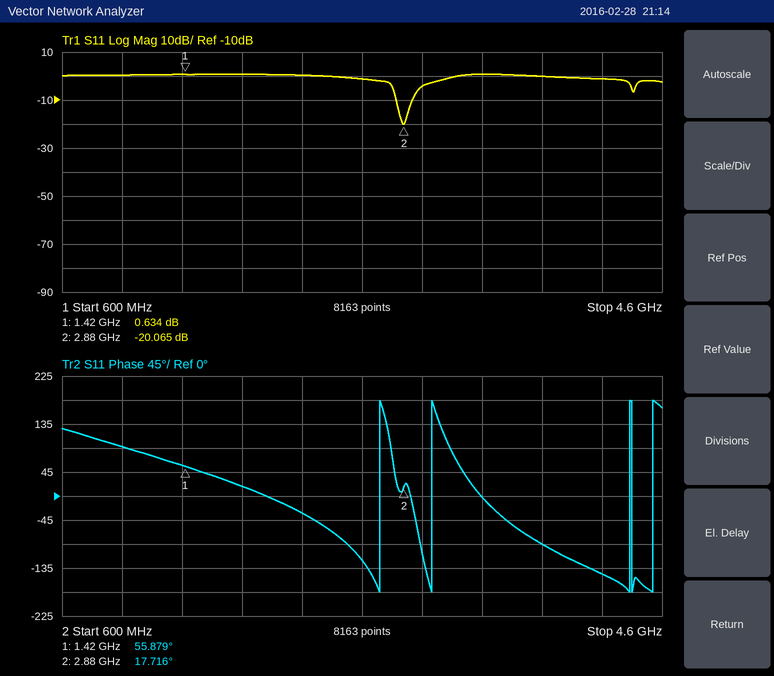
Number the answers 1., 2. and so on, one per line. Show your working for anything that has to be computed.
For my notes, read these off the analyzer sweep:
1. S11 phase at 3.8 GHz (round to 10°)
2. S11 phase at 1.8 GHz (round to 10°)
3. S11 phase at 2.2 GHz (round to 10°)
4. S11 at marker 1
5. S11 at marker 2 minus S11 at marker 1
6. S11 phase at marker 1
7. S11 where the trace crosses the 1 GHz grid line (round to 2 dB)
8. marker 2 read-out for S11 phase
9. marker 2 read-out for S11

1. -90°
2. 20°
3. -30°
4. 0.634 dB
5. -20.065 − (0.634) = -20.699 dB
6. 55.879°
7. 0 dB
8. 17.716°
9. -20.065 dB
